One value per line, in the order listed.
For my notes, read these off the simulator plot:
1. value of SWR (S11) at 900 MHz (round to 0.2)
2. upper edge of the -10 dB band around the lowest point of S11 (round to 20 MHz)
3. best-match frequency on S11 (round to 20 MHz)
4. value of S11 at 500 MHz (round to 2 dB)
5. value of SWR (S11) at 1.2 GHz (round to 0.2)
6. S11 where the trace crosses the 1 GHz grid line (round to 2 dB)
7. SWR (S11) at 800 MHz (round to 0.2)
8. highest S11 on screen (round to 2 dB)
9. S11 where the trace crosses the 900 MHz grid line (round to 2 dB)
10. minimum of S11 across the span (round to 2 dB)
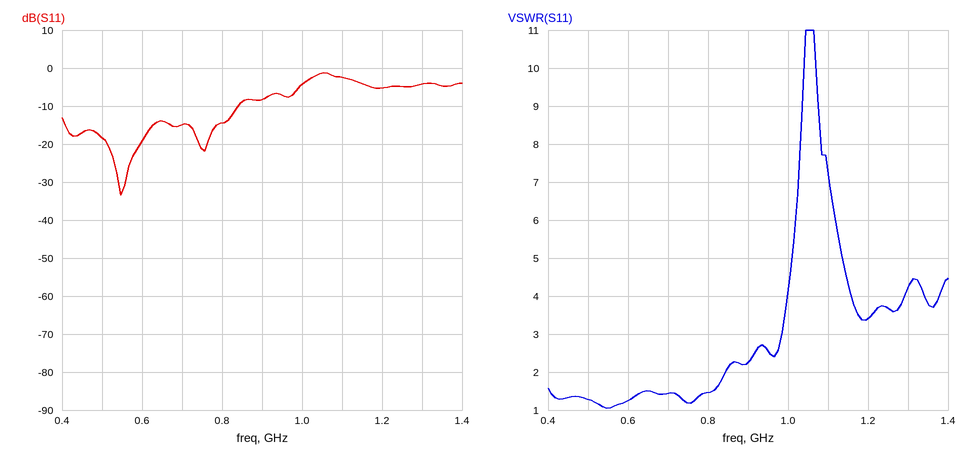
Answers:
2.2
840 MHz
540 MHz
-18 dB
3.4
-4 dB
1.4
-2 dB
-8 dB
-34 dB
